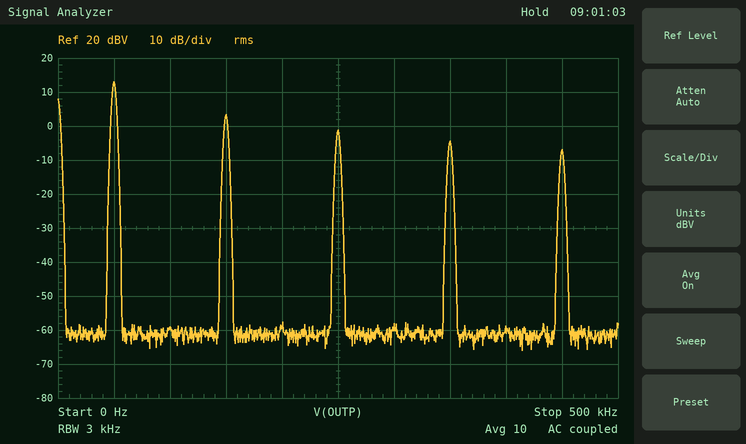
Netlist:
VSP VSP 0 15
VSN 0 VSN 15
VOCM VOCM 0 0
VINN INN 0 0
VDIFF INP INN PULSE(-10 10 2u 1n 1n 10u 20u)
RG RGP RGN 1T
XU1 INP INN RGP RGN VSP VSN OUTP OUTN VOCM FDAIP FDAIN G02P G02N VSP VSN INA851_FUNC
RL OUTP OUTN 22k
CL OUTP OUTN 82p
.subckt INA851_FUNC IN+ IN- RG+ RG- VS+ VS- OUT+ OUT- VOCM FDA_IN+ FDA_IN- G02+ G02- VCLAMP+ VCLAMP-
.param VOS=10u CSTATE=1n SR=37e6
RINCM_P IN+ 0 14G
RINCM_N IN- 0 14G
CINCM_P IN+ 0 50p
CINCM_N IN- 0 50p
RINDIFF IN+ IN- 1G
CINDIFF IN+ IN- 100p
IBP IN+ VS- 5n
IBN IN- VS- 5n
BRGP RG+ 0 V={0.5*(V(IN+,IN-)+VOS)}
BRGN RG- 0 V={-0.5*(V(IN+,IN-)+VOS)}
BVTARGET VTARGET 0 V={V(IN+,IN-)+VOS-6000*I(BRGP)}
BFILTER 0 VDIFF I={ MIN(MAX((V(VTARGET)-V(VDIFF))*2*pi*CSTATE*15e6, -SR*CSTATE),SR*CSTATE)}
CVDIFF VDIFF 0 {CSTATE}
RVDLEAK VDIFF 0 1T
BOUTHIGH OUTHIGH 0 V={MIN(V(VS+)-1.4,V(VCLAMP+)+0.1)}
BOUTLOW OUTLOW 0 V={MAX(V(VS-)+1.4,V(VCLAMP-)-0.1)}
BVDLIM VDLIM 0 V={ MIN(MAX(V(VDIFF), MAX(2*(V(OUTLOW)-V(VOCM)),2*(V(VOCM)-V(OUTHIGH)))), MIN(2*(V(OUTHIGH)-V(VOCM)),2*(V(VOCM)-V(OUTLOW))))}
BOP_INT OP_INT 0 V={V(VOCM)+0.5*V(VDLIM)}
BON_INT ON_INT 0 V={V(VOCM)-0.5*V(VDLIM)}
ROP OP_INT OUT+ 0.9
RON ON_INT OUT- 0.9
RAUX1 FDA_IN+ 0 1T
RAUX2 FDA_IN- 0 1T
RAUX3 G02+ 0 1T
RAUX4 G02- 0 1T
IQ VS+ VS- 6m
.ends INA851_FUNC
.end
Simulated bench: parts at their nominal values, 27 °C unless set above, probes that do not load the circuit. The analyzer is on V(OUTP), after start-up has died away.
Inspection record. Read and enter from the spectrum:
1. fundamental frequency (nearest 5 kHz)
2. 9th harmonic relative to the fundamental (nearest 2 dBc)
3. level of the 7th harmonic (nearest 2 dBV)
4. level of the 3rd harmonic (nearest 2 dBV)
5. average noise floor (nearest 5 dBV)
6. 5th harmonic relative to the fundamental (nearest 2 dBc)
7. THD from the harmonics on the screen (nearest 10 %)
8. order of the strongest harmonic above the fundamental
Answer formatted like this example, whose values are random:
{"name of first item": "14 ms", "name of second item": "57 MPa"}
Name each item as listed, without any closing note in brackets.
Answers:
{"fundamental frequency": "50 kHz", "9th harmonic relative to the fundamental": "-20 dBc", "level of the 7th harmonic": "-4 dBV", "level of the 3rd harmonic": "4 dBV", "average noise floor": "-60 dBV", "5th harmonic relative to the fundamental": "-14 dBc", "THD from the harmonics on the screen": "40 %", "order of the strongest harmonic above the fundamental": "3"}
